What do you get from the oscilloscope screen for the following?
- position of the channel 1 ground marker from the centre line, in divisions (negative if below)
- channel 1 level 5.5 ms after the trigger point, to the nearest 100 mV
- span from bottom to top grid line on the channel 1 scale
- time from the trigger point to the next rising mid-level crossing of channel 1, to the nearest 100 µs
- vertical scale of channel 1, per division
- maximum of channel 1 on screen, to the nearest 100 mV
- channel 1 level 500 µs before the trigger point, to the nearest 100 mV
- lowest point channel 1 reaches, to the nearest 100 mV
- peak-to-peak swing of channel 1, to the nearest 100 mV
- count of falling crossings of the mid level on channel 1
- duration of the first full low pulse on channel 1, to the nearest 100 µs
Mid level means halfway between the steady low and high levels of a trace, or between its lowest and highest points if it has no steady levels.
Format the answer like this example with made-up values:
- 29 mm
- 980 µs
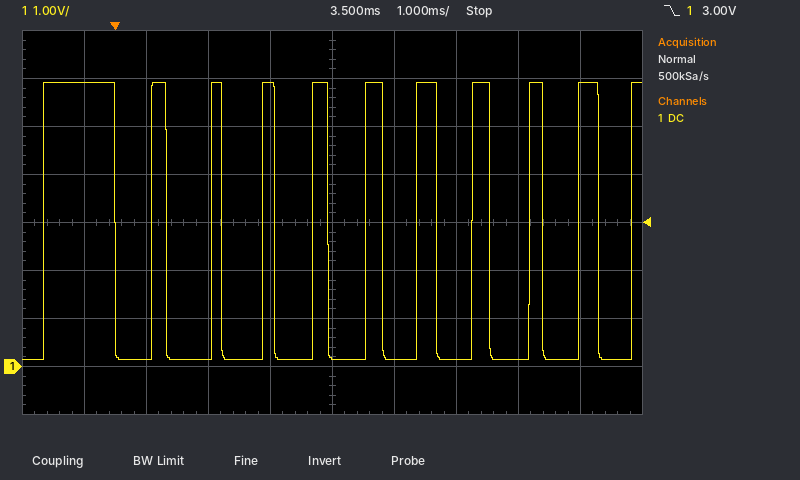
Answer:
- -3.0 div
- 100 mV
- 8 V
- 600 µs
- 1 V
- 5.9 V
- 5.9 V
- 100 mV
- 5.8 V
- 10
- 600 µs
